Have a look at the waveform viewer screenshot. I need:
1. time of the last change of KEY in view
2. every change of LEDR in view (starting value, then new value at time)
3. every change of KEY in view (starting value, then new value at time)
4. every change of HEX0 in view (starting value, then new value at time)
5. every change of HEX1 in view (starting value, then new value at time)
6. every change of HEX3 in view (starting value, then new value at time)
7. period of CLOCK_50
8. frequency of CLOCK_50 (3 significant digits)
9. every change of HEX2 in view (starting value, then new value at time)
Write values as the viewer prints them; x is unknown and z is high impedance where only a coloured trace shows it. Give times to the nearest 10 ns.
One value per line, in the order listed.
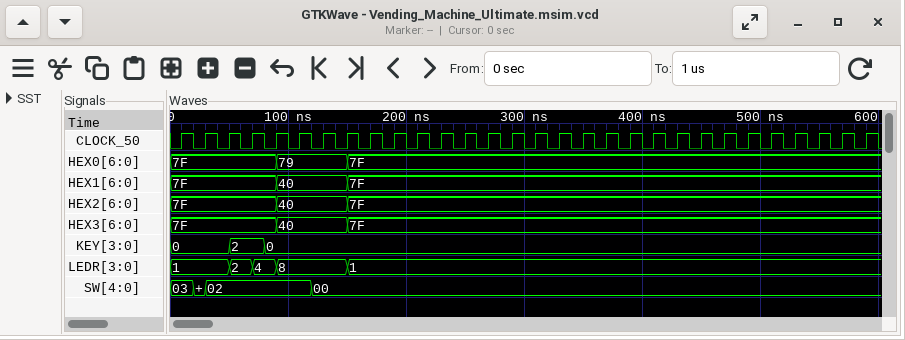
80 ns
1, 2 at 50 ns, 4 at 70 ns, 8 at 90 ns, 1 at 150 ns
0, 2 at 50 ns, 0 at 80 ns
7F, 79 at 90 ns, 7F at 150 ns
7F, 40 at 90 ns, 7F at 150 ns
7F, 40 at 90 ns, 7F at 150 ns
20 ns
50.0 MHz
7F, 40 at 90 ns, 7F at 150 ns
